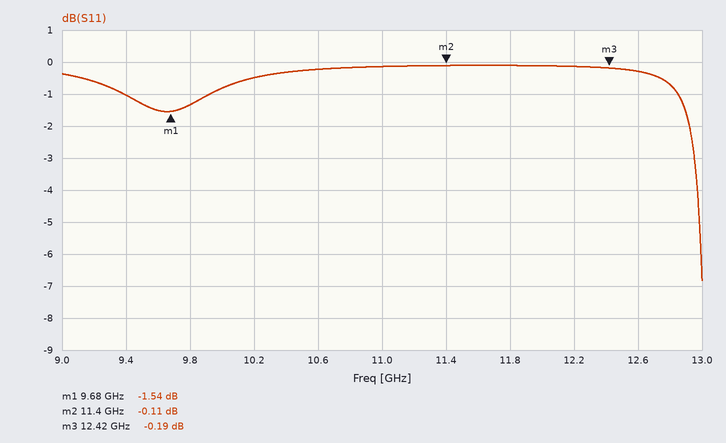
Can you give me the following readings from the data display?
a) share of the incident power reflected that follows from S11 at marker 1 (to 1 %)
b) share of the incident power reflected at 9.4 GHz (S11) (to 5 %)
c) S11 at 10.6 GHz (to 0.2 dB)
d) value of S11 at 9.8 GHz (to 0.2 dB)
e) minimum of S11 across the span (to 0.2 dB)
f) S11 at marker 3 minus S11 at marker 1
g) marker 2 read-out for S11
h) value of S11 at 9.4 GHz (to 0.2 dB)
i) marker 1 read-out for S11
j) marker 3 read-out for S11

70 %
80 %
-0.2 dB
-1.4 dB
-6.8 dB
1.35 dB
-0.11 dB
-1.0 dB
-1.54 dB
-0.19 dB
